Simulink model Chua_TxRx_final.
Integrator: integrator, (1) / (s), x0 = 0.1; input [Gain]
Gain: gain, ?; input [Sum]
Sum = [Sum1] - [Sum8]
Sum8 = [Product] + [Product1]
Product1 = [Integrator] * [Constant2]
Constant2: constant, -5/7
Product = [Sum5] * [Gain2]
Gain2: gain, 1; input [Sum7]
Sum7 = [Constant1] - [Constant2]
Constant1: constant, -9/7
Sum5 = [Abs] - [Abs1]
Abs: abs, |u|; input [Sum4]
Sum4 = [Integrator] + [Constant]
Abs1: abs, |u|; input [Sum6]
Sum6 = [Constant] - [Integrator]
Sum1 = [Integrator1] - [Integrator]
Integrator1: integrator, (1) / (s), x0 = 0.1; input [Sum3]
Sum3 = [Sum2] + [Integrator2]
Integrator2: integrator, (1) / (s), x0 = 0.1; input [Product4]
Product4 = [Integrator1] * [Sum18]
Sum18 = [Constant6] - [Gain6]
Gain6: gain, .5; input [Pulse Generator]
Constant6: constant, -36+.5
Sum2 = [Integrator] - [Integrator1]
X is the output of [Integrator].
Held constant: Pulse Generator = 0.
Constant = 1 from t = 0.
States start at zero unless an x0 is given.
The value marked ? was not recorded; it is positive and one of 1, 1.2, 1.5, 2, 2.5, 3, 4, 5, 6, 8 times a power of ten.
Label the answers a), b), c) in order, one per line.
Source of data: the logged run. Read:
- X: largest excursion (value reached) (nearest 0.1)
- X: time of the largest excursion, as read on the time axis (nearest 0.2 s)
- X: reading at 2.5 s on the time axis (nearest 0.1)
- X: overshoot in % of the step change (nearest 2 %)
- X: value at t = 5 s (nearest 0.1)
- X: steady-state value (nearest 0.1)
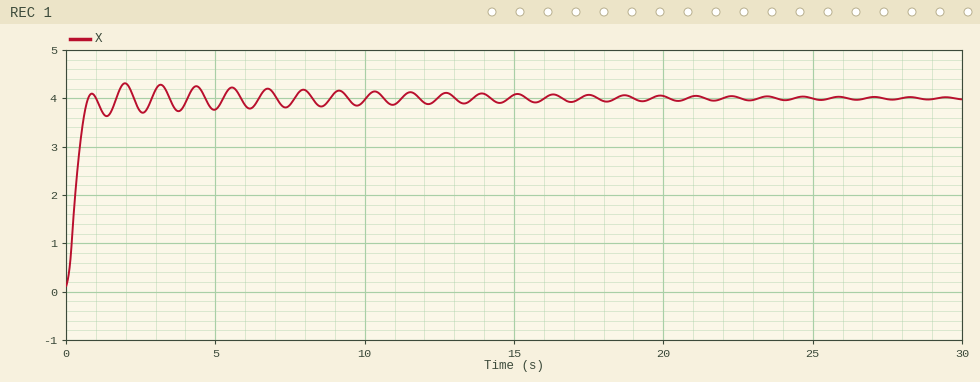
a) 4.3
b) 2.0 s
c) 3.7
d) 8 %
e) 3.8
f) 4.0
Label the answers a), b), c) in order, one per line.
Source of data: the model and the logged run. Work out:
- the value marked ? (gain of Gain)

a) 10
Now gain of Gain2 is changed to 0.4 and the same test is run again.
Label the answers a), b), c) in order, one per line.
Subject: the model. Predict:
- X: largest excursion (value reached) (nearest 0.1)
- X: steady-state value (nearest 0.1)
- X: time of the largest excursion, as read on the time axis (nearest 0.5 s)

a) 1.7
b) 1.6
c) 2.5 s
